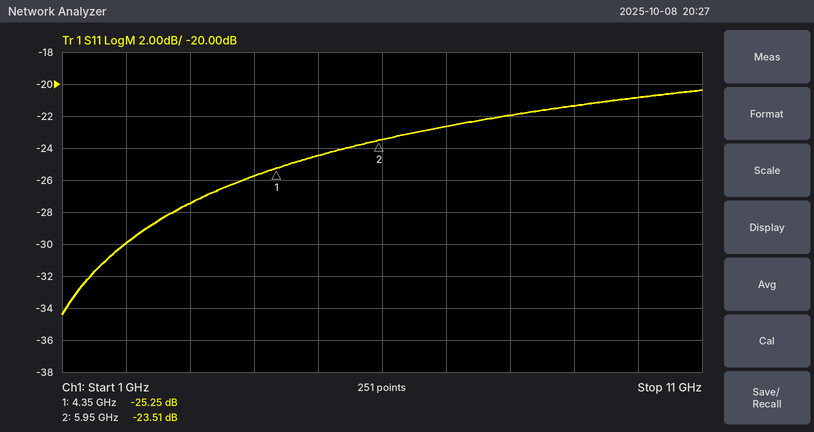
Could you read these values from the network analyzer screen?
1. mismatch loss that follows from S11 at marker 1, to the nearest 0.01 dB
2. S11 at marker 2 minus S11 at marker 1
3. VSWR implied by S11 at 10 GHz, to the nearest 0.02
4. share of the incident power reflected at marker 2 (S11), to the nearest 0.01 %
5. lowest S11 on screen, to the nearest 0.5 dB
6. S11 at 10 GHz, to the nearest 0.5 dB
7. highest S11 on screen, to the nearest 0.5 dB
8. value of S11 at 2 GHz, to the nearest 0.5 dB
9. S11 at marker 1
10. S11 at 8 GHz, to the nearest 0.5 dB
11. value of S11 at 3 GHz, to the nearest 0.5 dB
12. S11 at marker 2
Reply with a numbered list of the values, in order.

1. 0.01 dB
2. 1.74 dB
3. 1.20
4. 0.45 %
5. -34.5 dB
6. -21.0 dB
7. -20.5 dB
8. -30.0 dB
9. -25.25 dB
10. -22.0 dB
11. -27.5 dB
12. -23.51 dB
